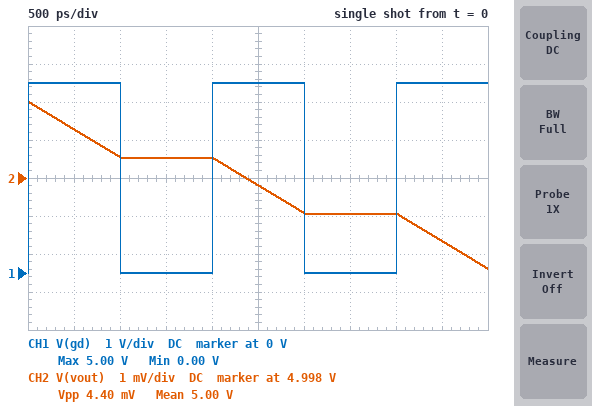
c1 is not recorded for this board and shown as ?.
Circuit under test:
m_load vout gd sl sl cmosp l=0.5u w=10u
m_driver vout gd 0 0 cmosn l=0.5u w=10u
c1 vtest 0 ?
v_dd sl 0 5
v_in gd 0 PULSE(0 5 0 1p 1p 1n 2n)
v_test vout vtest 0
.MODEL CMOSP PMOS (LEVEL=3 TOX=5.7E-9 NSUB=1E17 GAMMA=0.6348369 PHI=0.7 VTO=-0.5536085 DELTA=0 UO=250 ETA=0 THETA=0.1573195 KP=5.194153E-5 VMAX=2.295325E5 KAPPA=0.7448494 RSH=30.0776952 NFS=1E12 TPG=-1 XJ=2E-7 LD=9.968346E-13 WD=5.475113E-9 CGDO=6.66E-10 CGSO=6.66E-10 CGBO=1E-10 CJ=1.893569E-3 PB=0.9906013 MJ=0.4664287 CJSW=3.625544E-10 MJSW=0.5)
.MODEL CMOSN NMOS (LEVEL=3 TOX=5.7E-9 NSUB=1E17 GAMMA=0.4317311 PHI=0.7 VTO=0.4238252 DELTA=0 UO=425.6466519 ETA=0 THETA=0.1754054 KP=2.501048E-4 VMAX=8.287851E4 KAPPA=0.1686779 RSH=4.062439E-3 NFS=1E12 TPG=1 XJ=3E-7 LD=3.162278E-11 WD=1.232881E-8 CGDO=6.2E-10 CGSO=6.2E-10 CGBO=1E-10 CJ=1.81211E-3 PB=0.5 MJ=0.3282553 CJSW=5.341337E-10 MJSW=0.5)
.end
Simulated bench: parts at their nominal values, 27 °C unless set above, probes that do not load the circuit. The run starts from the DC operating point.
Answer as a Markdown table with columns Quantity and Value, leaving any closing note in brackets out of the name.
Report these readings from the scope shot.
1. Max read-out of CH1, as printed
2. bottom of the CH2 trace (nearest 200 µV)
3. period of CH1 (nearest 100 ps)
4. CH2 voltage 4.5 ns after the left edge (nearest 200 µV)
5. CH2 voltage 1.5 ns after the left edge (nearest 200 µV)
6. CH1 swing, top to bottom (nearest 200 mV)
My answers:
| Quantity | Value |
|---|---|
| Max read-out of CH1, as printed | 5.00 V |
| bottom of the CH2 trace | 4.9956 V |
| period of CH1 | 2.0 ns |
| CH2 voltage 4.5 ns after the left edge | 4.9964 V |
| CH2 voltage 1.5 ns after the left edge | 4.9986 V |
| CH1 swing, top to bottom | 5.0 V |
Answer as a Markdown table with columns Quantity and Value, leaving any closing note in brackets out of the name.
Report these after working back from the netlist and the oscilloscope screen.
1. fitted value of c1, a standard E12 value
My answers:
| Quantity | Value |
|---|---|
| fitted value of c1, a standard E12 value | 6.8 nF |
